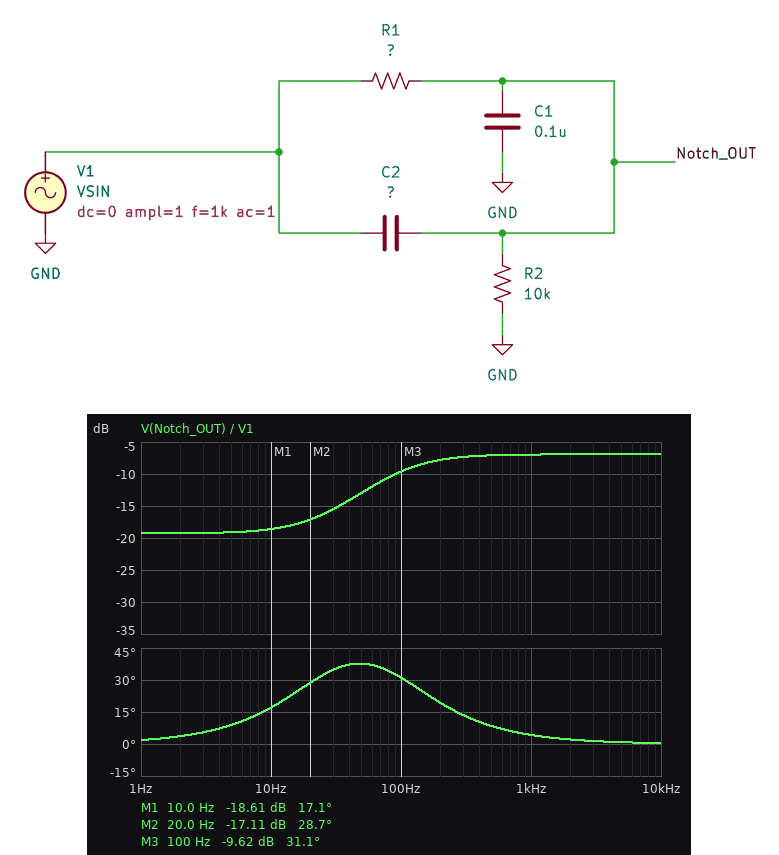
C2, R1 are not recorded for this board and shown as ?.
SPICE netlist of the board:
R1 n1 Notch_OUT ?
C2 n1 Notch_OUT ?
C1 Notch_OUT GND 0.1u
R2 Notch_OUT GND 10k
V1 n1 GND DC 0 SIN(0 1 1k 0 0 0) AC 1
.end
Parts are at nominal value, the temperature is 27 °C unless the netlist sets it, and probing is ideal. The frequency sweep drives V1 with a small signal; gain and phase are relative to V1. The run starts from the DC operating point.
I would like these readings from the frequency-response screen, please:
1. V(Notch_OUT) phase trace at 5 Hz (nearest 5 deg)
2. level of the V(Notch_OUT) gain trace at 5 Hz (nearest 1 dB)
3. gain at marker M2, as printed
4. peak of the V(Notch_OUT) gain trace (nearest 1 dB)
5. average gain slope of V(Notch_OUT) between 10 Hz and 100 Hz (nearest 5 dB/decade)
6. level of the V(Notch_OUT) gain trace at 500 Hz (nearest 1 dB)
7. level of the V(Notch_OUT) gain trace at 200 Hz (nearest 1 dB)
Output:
10 deg
-19 dB
-17.11 dB
-7 dB
10 dB/decade
-7 dB
-8 dB
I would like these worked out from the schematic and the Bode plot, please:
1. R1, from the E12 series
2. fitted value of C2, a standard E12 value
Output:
82 kΩ
82 nF
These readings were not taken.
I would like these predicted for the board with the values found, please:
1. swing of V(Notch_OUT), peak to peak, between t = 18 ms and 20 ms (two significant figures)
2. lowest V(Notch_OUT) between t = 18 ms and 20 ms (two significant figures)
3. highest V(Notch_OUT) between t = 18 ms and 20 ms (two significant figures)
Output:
900 mV
-450 mV
450 mV
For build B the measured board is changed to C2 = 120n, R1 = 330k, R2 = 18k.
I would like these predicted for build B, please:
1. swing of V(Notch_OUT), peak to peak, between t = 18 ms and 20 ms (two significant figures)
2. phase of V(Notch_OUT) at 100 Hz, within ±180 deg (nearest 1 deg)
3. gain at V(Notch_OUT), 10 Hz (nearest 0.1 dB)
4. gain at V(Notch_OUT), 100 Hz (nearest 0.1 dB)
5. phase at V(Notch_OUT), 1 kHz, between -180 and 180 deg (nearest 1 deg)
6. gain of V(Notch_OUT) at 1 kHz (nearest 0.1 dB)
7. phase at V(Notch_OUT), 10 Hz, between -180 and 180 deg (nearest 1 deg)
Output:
1.1 V
21 deg
-17.4 dB
-6.0 dB
2 deg
-5.3 dB
55 deg
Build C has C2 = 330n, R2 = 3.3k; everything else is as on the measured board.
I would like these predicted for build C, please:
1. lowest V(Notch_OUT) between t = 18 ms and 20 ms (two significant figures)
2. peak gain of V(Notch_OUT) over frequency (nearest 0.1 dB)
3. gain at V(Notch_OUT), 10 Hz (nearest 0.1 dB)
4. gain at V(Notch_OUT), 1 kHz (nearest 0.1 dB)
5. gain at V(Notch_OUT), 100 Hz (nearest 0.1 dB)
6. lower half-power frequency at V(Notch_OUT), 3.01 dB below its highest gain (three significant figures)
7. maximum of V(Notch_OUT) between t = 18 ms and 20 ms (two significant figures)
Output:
-760 mV
-2.3 dB
-22.4 dB
-2.4 dB
-6.0 dB
116 Hz
760 mV
